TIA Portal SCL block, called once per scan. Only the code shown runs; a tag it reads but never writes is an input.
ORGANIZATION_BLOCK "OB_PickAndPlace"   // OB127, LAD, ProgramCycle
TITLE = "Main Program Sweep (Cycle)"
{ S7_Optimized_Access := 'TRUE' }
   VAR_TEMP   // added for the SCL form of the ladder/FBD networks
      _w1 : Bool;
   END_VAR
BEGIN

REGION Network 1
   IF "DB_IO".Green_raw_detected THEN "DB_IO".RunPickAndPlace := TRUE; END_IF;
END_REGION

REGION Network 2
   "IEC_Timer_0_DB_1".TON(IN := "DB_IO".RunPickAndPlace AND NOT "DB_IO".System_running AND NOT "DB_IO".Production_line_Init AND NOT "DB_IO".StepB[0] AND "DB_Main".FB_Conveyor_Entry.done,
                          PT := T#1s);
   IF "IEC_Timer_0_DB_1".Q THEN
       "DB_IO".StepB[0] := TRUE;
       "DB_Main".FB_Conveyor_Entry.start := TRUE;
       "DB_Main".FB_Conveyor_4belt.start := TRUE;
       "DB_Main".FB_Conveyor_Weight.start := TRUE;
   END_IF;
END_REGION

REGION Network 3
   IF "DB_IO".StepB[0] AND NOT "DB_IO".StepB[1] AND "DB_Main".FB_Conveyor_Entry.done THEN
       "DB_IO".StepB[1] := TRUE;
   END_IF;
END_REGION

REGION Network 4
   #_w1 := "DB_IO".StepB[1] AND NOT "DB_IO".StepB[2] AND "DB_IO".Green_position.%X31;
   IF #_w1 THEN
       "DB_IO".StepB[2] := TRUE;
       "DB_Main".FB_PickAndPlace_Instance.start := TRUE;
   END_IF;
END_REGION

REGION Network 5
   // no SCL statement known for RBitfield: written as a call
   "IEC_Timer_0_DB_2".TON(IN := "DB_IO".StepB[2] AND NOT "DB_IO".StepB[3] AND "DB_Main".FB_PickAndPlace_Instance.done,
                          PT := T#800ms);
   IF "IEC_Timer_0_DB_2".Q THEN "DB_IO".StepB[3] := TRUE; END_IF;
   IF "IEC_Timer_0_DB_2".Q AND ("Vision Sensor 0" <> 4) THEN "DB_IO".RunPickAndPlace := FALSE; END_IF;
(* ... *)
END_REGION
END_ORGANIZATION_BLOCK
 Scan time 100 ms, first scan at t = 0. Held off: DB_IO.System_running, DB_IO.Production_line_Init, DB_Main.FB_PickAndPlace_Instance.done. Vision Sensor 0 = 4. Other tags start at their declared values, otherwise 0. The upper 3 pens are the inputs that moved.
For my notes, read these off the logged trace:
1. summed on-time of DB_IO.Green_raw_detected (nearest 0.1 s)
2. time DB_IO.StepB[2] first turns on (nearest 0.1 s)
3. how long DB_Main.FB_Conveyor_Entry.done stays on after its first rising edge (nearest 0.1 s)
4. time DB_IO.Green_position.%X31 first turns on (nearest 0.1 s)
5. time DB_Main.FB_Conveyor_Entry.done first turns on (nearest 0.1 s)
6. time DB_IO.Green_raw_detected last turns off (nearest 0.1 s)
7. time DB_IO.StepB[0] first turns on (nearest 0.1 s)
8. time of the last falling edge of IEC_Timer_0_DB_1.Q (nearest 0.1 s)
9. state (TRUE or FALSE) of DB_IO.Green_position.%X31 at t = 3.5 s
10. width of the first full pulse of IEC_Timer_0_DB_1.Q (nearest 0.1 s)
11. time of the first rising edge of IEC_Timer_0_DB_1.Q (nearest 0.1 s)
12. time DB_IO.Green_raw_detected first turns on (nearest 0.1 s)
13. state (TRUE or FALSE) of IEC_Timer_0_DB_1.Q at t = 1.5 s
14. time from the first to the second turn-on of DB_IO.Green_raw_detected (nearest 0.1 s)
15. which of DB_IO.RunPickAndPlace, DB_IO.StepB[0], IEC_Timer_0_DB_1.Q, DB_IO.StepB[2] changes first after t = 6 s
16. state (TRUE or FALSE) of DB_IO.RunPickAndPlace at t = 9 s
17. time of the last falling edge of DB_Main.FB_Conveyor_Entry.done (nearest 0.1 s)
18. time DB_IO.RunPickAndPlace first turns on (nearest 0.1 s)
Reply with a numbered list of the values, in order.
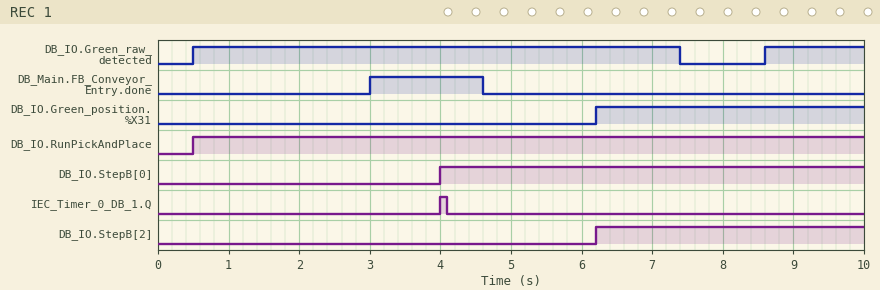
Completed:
1. 8.3 s
2. 6.2 s
3. 1.6 s
4. 6.2 s
5. 3.0 s
6. 7.4 s
7. 4.0 s
8. 4.1 s
9. FALSE
10. 0.1 s
11. 4.0 s
12. 0.5 s
13. FALSE
14. 8.1 s
15. DB_IO.StepB[2]
16. TRUE
17. 4.6 s
18. 0.5 s
